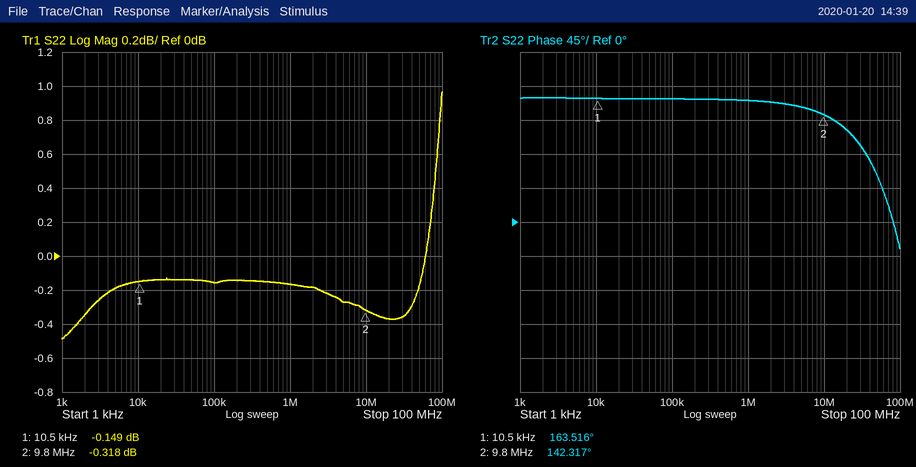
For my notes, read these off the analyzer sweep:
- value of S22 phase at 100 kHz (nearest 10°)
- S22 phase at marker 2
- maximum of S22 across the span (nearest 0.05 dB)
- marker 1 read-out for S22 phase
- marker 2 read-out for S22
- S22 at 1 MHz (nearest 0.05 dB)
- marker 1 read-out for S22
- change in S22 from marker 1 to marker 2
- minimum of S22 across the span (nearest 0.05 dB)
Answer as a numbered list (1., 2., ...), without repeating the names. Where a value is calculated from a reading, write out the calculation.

1. 160°
2. 142.317°
3. 0.95 dB
4. 163.516°
5. -0.318 dB
6. -0.15 dB
7. -0.149 dB
8. -0.318 − (-0.149) = -0.169 dB
9. -0.50 dB
